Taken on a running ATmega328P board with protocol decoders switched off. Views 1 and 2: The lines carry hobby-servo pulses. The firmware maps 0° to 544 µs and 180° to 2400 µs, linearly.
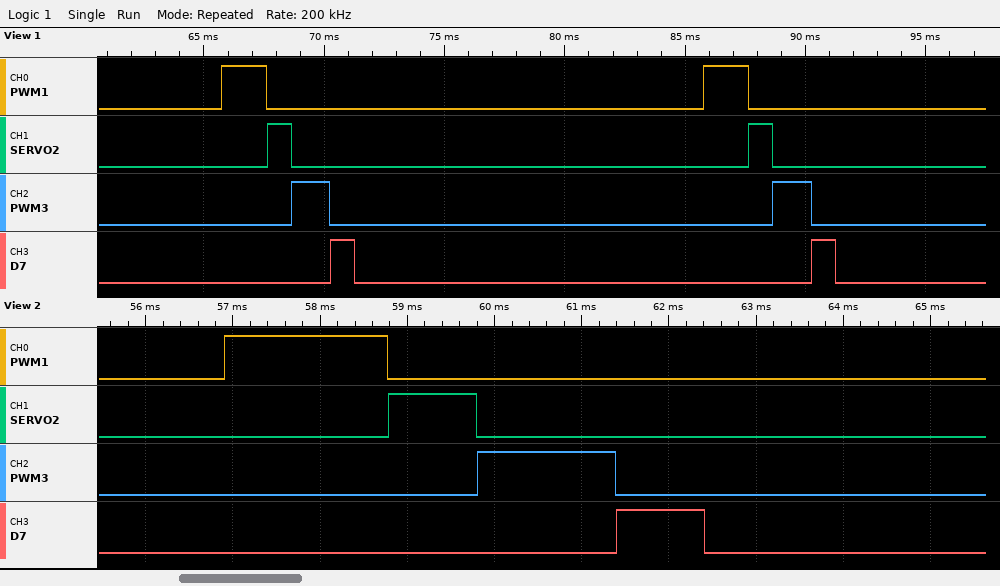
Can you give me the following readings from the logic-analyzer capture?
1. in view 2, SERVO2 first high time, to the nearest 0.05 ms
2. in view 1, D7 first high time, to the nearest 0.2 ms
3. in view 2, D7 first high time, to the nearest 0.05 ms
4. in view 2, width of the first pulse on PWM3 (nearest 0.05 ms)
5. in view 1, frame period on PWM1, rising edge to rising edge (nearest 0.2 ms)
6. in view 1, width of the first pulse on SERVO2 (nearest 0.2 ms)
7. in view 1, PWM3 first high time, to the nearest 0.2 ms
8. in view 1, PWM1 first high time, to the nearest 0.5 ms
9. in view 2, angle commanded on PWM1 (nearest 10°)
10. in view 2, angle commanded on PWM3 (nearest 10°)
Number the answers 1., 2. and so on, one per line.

1. 1.00 ms
2. 1.0 ms
3. 1.00 ms
4. 1.60 ms
5. 20.0 ms
6. 1.0 ms
7. 1.6 ms
8. 2.0 ms
9. 130°
10. 100°
